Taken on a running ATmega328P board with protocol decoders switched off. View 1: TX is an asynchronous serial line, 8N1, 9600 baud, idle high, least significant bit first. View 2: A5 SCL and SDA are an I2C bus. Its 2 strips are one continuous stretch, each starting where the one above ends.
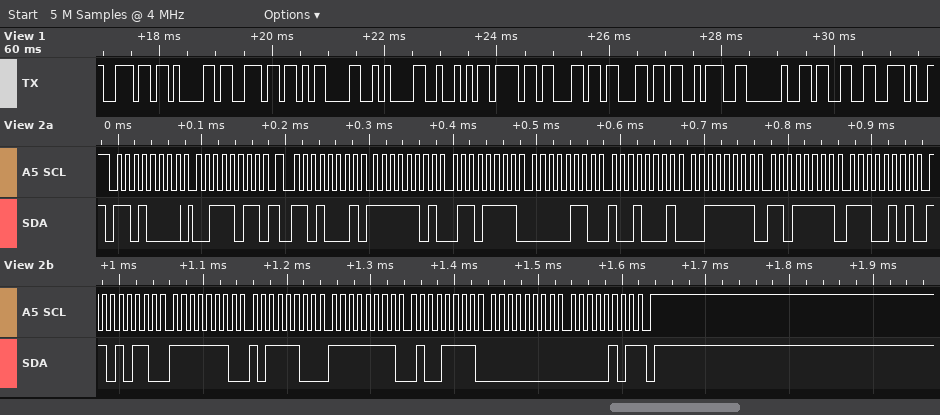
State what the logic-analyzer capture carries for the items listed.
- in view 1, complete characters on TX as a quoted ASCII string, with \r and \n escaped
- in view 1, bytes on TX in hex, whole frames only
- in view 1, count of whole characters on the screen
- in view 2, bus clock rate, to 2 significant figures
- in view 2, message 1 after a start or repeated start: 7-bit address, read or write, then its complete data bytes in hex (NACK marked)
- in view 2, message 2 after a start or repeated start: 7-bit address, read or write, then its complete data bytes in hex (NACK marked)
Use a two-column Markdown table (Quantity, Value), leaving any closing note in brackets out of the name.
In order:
| Quantity | Value |
|---|---|
| in view 1, complete characters on TX as a quoted ASCII string, with \r and \n escaped | "nan\r\nRoll: 3." |
| in view 1, bytes on TX in hex, whole frames only | 6E 61 6E 0D 0A 52 6F 6C 6C 3A 20 33 2E |
| in view 1, count of whole characters on the screen | 13 |
| in view 2, bus clock rate, to 2 significant figures | 100 kHz |
| in view 2, message 1 after a start or repeated start: 7-bit address, read or write, then its complete data bytes in hex | 0x68 write: 3B |
| in view 2, message 2 after a start or repeated start: 7-bit address, read or write, then its complete data bytes in hex | 0x68 read: FD 6F 06 91 3F DF E5 D6 FE BC FF 4F 00 05 NACK |
